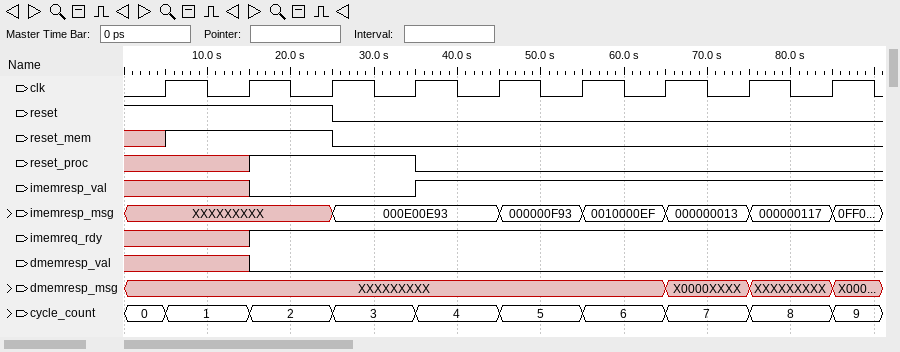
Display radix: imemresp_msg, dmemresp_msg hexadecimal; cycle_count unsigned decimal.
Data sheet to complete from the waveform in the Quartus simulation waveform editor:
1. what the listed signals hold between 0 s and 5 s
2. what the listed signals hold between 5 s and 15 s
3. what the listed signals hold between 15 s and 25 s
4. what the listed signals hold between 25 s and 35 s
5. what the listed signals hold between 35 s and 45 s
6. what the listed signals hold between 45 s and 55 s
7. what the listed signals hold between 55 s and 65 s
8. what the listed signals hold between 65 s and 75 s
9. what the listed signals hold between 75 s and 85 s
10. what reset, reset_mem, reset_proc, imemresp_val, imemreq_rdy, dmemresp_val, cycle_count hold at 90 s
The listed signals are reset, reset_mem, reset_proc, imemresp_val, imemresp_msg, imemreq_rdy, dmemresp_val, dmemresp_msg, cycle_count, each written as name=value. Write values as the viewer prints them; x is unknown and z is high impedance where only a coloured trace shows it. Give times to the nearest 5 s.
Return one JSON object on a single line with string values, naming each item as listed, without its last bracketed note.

{"what the listed signals hold between 0 s and 5 s": "reset=1, reset_mem=x, reset_proc=x, imemresp_val=x, imemresp_msg=XXXXXXXXX, imemreq_rdy=x, dmemresp_val=x, dmemresp_msg=XXXXXXXXX, cycle_count=0", "what the listed signals hold between 5 s and 15 s": "reset=1, reset_mem=1, reset_proc=x, imemresp_val=x, imemresp_msg=XXXXXXXXX, imemreq_rdy=x, dmemresp_val=x, dmemresp_msg=XXXXXXXXX, cycle_count=1", "what the listed signals hold between 15 s and 25 s": "reset=1, reset_mem=1, reset_proc=1, imemresp_val=0, imemresp_msg=XXXXXXXXX, imemreq_rdy=1, dmemresp_val=0, dmemresp_msg=XXXXXXXXX, cycle_count=2", "what the listed signals hold between 25 s and 35 s": "reset=0, reset_mem=0, reset_proc=1, imemresp_val=0, imemresp_msg=000E00E93, imemreq_rdy=1, dmemresp_val=0, dmemresp_msg=XXXXXXXXX, cycle_count=3", "what the listed signals hold between 35 s and 45 s": "reset=0, reset_mem=0, reset_proc=0, imemresp_val=1, imemresp_msg=000E00E93, imemreq_rdy=1, dmemresp_val=0, dmemresp_msg=XXXXXXXXX, cycle_count=4", "what the listed signals hold between 45 s and 55 s": "reset=0, reset_mem=0, reset_proc=0, imemresp_val=1, imemresp_msg=000000F93, imemreq_rdy=1, dmemresp_val=0, dmemresp_msg=XXXXXXXXX, cycle_count=5", "what the listed signals hold between 55 s and 65 s": "reset=0, reset_mem=0, reset_proc=0, imemresp_val=1, imemresp_msg=0010000EF, imemreq_rdy=1, dmemresp_val=0, dmemresp_msg=XXXXXXXXX, cycle_count=6", "what the listed signals hold between 65 s and 75 s": "reset=0, reset_mem=0, reset_proc=0, imemresp_val=1, imemresp_msg=000000013, imemreq_rdy=1, dmemresp_val=0, dmemresp_msg=X0000XXXX, cycle_count=7", "what the listed signals hold between 75 s and 85 s": "reset=0, reset_mem=0, reset_proc=0, imemresp_val=1, imemresp_msg=000000117, imemreq_rdy=1, dmemresp_val=0, dmemresp_msg=XXXXXXXXX, cycle_count=8", "what reset, reset_mem, reset_proc, imemresp_val, imemreq_rdy, dmemresp_val, cycle_count hold at 90 s": "reset=0, reset_mem=0, reset_proc=0, imemresp_val=1, imemreq_rdy=1, dmemresp_val=0, cycle_count=9"}
